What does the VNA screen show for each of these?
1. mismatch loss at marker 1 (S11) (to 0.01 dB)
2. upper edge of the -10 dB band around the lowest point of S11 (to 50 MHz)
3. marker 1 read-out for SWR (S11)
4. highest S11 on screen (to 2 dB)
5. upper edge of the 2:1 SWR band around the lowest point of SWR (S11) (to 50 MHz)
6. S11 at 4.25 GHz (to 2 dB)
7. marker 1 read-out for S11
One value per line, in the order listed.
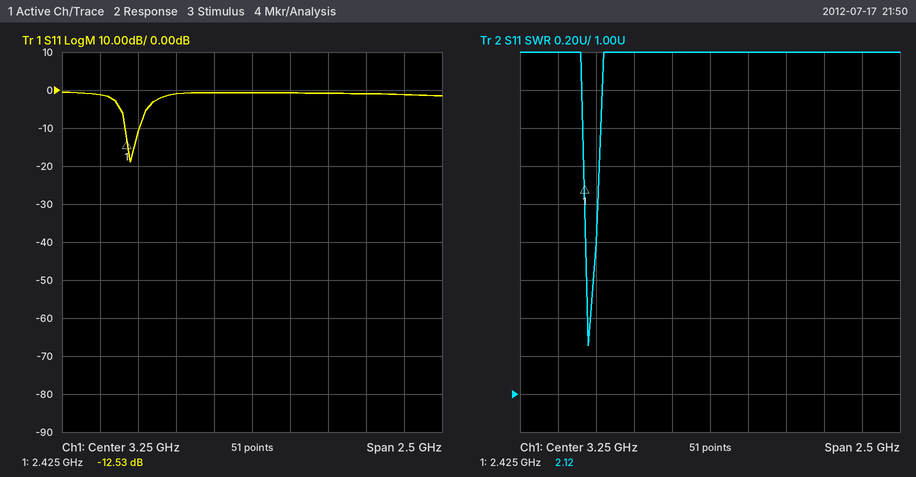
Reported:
0.25 dB
2.50 GHz
2.12
0 dB
2.50 GHz
-2 dB
-12.53 dB
